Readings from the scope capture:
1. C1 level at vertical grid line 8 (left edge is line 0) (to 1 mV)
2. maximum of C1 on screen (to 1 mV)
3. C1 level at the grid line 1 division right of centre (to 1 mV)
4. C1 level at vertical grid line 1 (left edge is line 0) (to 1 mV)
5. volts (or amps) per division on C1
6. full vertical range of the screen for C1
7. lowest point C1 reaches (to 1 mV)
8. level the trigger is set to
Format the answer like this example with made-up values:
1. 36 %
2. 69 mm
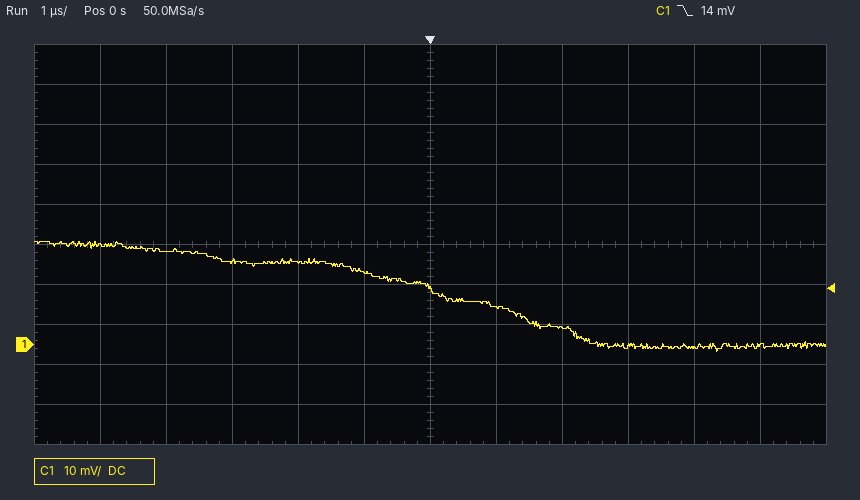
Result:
1. 4 mV
2. 26 mV
3. 9 mV
4. 25 mV
5. 10 mV
6. 100 mV
7. -2 mV
8. 14 mV
